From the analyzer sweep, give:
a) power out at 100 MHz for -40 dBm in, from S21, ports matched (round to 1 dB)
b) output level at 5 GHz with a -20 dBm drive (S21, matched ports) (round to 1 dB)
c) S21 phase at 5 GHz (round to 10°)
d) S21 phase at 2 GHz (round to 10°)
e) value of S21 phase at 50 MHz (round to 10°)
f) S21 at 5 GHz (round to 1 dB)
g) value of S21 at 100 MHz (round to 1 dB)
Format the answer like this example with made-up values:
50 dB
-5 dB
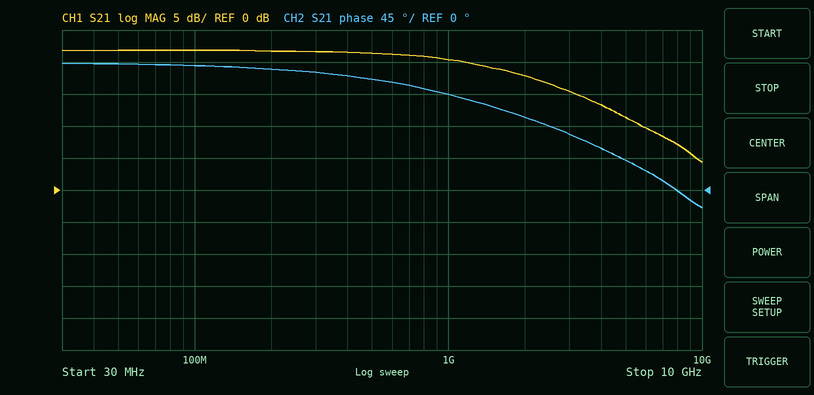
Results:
-18 dBm
-9 dBm
40°
100°
180°
11 dB
22 dB
